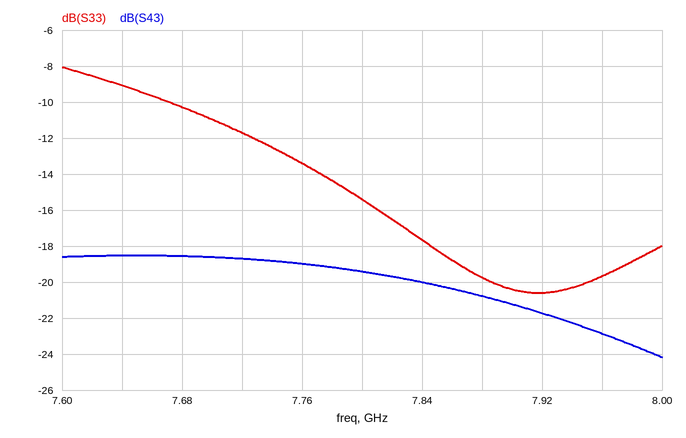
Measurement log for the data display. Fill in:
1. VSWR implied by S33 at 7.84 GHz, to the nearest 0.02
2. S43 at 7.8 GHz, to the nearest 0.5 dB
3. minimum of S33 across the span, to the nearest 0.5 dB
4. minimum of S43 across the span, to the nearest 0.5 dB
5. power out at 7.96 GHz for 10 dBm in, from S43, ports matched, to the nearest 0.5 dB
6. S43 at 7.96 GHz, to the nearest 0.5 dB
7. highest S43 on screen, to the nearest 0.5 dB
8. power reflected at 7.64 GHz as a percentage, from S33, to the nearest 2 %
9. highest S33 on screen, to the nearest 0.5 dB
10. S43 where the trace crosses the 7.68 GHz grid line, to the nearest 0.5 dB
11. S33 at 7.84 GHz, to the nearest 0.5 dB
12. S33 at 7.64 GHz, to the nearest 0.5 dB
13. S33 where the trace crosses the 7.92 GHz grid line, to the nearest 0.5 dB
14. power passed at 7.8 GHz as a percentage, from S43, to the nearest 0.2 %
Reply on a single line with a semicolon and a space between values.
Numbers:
1.30; -19.5 dB; -20.5 dB; -24.0 dB; -13.0 dBm; -23.0 dB; -18.5 dB; 12 %; -8.0 dB; -18.5 dB; -17.5 dB; -9.0 dB; -20.5 dB; 1.2 %
